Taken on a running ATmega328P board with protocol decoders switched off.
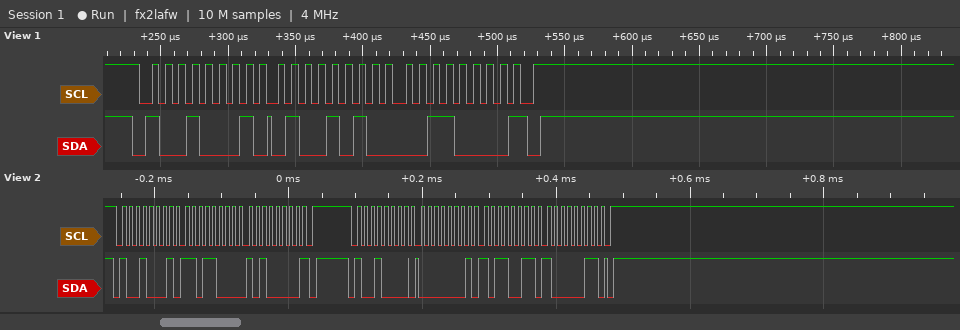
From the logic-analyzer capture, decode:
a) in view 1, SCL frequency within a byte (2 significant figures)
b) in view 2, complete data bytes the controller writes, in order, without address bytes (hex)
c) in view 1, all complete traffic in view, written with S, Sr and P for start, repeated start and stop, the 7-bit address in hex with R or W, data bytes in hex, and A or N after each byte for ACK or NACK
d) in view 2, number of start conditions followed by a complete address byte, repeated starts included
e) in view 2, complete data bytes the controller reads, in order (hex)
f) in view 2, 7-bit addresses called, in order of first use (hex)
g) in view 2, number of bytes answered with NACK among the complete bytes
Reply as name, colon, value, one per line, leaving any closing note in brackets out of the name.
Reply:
in view 1, SCL frequency within a byte: 100 kHz
in view 2, complete data bytes the controller writes, in order, without address bytes: 01 B3 83
in view 1, all complete traffic in view, written with S, Sr and P for start, repeated start and stop, the 7-bit address in hex with R or W, data bytes in hex, and A or N after each byte for ACK or NACK: S 48R A 4A A 30 N P
in view 2, number of start conditions followed by a complete address byte, repeated starts included: 2
in view 2, complete data bytes the controller reads, in order: D8 A0
in view 2, 7-bit addresses called, in order of first use: 0x48
in view 2, number of bytes answered with NACK among the complete bytes: 1
